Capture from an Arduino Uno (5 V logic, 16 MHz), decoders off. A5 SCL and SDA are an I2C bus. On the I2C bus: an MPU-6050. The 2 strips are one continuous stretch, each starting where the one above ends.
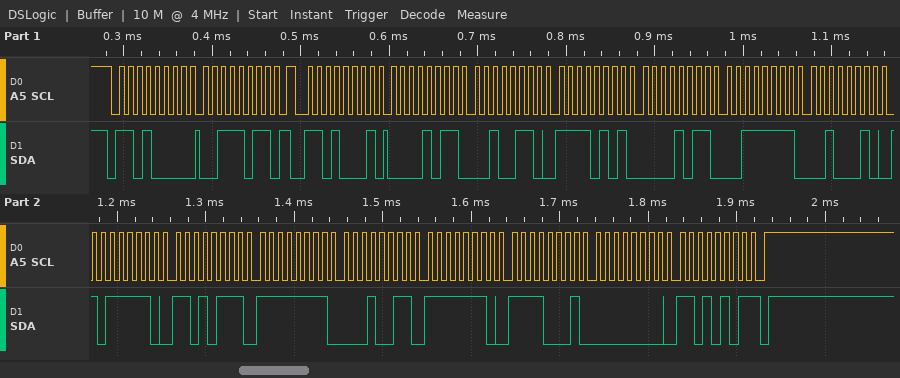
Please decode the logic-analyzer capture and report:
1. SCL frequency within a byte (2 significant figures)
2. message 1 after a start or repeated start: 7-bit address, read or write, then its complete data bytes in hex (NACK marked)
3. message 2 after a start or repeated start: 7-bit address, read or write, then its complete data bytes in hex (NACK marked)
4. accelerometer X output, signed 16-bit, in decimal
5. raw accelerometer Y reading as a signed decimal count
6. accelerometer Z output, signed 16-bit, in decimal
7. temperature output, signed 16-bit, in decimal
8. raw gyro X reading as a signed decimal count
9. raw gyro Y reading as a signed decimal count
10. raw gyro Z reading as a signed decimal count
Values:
100 kHz
0x68 write: 3B
0x68 read: 0B 26 F5 0B 3F 22 BE D7 FF 13 FE F1 00 D5 NACK
2854
-2805
16162
-16681
-237
-271
213
